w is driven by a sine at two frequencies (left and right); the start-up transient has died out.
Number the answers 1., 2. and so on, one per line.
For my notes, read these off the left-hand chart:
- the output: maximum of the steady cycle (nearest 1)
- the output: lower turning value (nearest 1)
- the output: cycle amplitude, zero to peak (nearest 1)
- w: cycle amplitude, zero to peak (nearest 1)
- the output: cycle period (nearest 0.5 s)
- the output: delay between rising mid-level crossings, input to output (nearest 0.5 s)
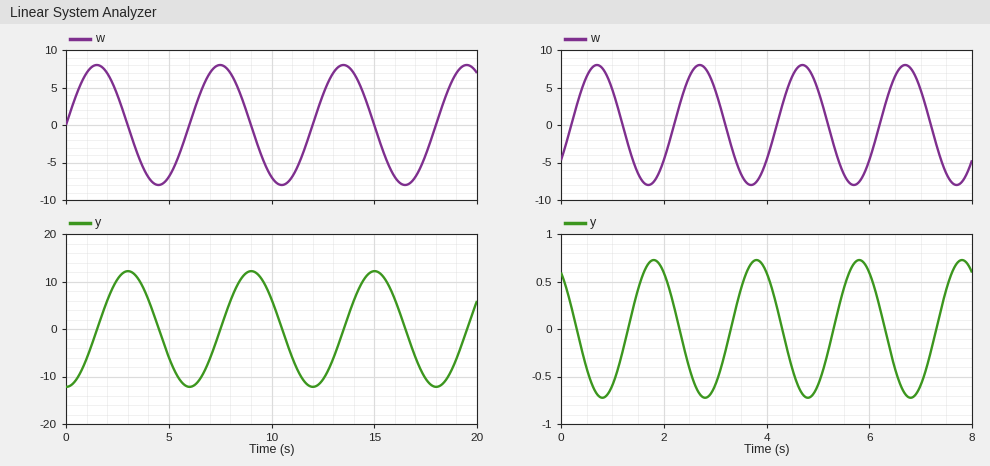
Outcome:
1. 12
2. -12
3. 12
4. 8
5. 6.0 s
6. 1.5 s
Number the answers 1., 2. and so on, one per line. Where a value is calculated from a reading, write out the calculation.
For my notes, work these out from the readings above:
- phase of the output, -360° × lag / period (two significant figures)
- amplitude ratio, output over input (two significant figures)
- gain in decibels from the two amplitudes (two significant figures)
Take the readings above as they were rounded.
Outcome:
1. -360 × 1.5 / 6 = -90°
2. 12 / 8 = 1.5
3. 20 log10(12 / 8) = 3.5 dB
